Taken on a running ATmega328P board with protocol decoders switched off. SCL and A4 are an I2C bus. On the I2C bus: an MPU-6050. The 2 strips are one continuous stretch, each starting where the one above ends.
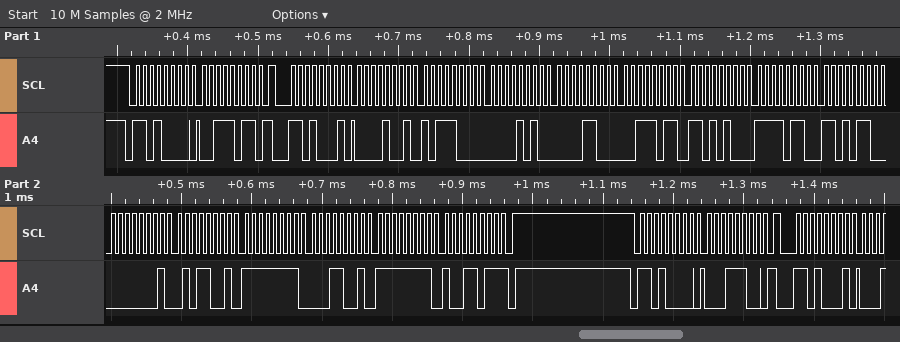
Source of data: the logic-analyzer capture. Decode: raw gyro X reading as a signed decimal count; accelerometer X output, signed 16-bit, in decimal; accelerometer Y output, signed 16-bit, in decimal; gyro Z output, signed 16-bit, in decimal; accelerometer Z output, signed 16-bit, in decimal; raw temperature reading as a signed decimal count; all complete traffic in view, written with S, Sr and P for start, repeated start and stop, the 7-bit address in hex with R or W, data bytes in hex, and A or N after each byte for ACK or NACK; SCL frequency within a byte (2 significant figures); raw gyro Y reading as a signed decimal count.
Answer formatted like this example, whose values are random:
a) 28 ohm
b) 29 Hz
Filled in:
a) 345
b) 2488
c) 2572
d) -101
e) 15316
f) -2346
g) S 68W A 3B A Sr 68R A 09 A B8 A 0A A 0C A 3B A D4 A F6 A D6 A 01 A 59 A FF A 19 A FF A 9B N P S 68W A 1C A Sr 68R A
h) 100 kHz
i) -231
